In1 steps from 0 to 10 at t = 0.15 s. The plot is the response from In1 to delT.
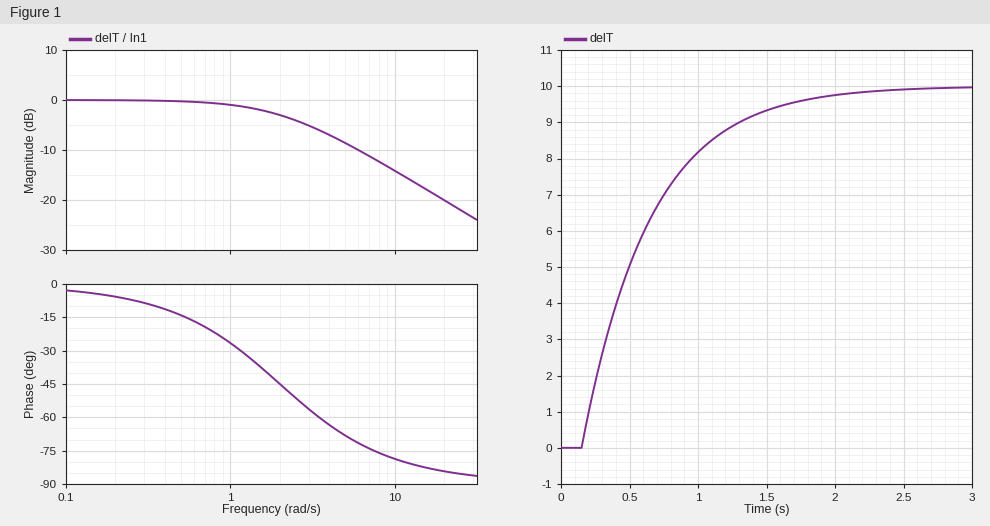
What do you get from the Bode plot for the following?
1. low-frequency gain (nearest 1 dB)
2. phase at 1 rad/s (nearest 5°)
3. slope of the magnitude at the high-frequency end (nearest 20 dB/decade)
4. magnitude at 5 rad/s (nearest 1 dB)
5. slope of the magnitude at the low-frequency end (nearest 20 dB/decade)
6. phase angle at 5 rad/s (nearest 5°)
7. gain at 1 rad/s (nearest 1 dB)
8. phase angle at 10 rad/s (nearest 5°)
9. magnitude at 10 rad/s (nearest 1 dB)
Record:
0 dB
-25°
-20 dB/decade
-9 dB
0 dB/decade
-70°
-1 dB
-80°
-14 dB
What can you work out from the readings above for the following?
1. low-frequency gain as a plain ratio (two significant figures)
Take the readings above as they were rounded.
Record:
1.0
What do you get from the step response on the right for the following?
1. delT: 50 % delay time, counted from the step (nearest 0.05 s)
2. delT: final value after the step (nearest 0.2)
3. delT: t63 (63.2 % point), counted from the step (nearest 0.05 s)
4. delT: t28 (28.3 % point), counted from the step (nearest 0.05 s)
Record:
0.35 s
10.0
0.50 s
0.15 s
